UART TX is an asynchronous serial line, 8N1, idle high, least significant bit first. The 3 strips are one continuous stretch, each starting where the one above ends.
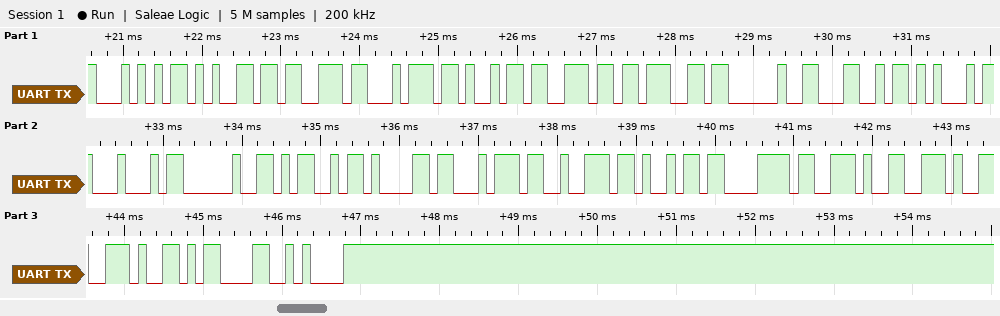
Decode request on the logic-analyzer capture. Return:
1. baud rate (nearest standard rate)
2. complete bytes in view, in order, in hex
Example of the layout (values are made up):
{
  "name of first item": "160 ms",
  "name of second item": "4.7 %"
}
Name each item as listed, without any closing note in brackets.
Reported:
{
  "baud rate": "9600 baud",
  "complete bytes in view, in order, in hex": "54 65 73 74 69 6E 67 20 4C 45 44 20 4D 61 74 72 69 78 2E 2E 2E 0D 0A"
}
